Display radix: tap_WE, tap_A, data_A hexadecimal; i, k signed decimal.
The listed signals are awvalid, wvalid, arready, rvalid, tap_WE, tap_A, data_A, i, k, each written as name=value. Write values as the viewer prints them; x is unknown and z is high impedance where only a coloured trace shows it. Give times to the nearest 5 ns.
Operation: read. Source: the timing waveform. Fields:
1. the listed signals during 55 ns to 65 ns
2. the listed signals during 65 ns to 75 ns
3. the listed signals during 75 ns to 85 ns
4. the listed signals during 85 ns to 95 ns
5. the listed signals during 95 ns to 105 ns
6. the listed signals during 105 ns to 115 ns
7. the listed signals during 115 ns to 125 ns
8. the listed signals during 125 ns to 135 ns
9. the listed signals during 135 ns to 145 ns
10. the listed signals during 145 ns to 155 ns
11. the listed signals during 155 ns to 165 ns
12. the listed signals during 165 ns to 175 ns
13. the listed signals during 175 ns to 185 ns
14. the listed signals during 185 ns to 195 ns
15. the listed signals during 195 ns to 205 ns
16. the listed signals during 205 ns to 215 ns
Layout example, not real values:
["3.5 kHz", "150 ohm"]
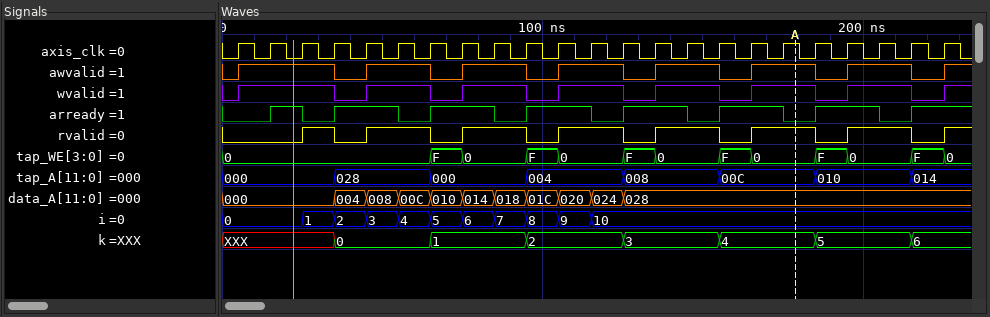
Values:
["awvalid=1, wvalid=1, arready=0, rvalid=1, tap_WE=0, tap_A=028, data_A=00C, i=4, k=0", "awvalid=0, wvalid=0, arready=1, rvalid=0, tap_WE=F, tap_A=000, data_A=010, i=5, k=1", "awvalid=1, wvalid=1, arready=1, rvalid=1, tap_WE=0, tap_A=000, data_A=014, i=6, k=1", "awvalid=1, wvalid=1, arready=0, rvalid=1, tap_WE=0, tap_A=000, data_A=018, i=7, k=1", "awvalid=0, wvalid=0, arready=1, rvalid=0, tap_WE=F, tap_A=004, data_A=01C, i=8, k=2", "awvalid=1, wvalid=1, arready=1, rvalid=1, tap_WE=0, tap_A=004, data_A=020, i=9, k=2", "awvalid=1, wvalid=1, arready=0, rvalid=1, tap_WE=0, tap_A=004, data_A=024, i=10, k=2", "awvalid=0, wvalid=0, arready=1, rvalid=0, tap_WE=F, tap_A=008, data_A=028, i=10, k=3", "awvalid=1, wvalid=1, arready=1, rvalid=1, tap_WE=0, tap_A=008, data_A=028, i=10, k=3", "awvalid=1, wvalid=1, arready=0, rvalid=1, tap_WE=0, tap_A=008, data_A=028, i=10, k=3", "awvalid=0, wvalid=0, arready=1, rvalid=0, tap_WE=F, tap_A=00C, data_A=028, i=10, k=4", "awvalid=1, wvalid=1, arready=1, rvalid=1, tap_WE=0, tap_A=00C, data_A=028, i=10, k=4", "awvalid=1, wvalid=1, arready=0, rvalid=1, tap_WE=0, tap_A=00C, data_A=028, i=10, k=4", "awvalid=0, wvalid=0, arready=1, rvalid=0, tap_WE=F, tap_A=010, data_A=028, i=10, k=5", "awvalid=1, wvalid=1, arready=1, rvalid=1, tap_WE=0, tap_A=010, data_A=028, i=10, k=5", "awvalid=1, wvalid=1, arready=0, rvalid=1, tap_WE=0, tap_A=010, data_A=028, i=10, k=5"]
